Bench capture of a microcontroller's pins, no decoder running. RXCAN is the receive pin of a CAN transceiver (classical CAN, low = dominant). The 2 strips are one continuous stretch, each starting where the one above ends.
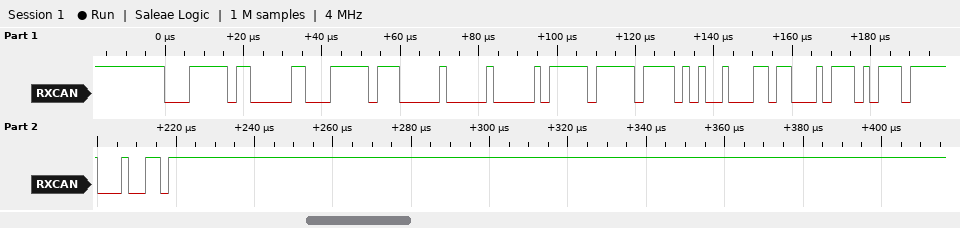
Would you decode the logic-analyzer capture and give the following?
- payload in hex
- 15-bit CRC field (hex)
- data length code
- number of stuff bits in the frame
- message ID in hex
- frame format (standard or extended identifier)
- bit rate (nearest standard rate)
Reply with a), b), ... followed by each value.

a) FF 00 00 FF FD 48 D8 BA
b) 0x77C9
c) 8
d) 9
e) 0x1FC
f) standard
g) 500 kbit/s
